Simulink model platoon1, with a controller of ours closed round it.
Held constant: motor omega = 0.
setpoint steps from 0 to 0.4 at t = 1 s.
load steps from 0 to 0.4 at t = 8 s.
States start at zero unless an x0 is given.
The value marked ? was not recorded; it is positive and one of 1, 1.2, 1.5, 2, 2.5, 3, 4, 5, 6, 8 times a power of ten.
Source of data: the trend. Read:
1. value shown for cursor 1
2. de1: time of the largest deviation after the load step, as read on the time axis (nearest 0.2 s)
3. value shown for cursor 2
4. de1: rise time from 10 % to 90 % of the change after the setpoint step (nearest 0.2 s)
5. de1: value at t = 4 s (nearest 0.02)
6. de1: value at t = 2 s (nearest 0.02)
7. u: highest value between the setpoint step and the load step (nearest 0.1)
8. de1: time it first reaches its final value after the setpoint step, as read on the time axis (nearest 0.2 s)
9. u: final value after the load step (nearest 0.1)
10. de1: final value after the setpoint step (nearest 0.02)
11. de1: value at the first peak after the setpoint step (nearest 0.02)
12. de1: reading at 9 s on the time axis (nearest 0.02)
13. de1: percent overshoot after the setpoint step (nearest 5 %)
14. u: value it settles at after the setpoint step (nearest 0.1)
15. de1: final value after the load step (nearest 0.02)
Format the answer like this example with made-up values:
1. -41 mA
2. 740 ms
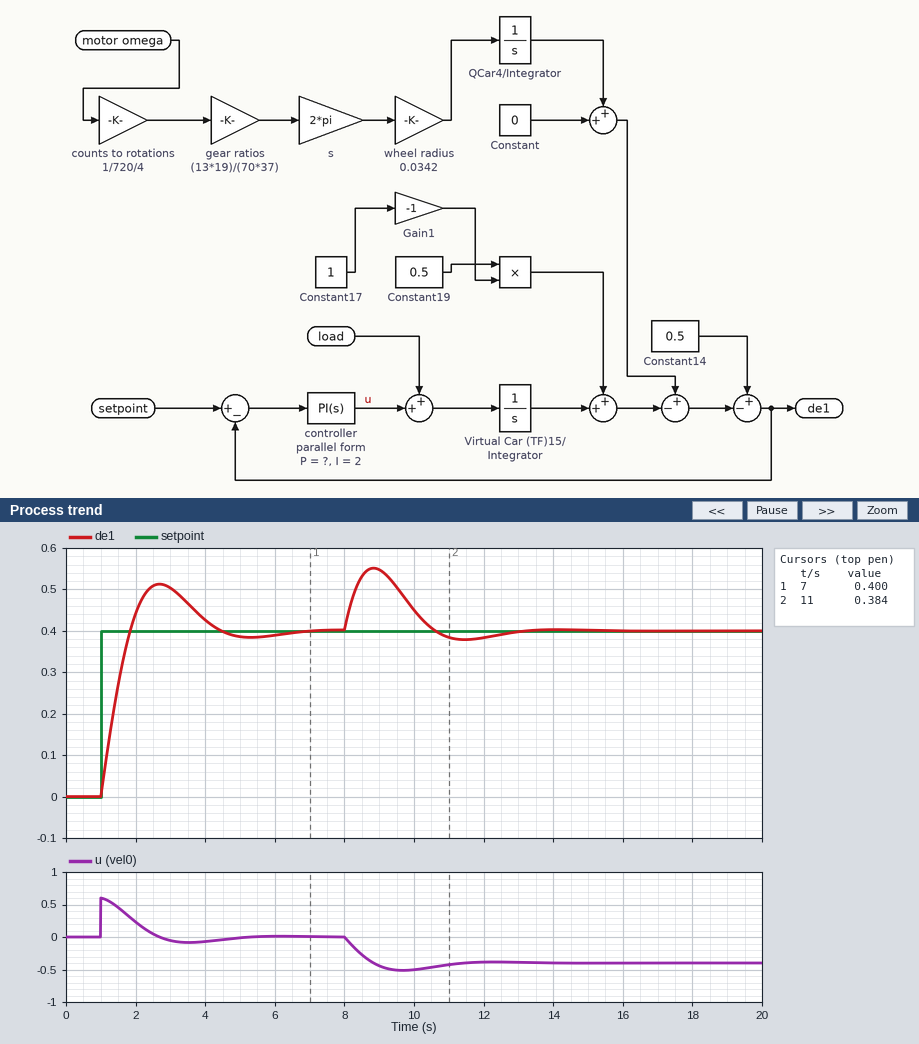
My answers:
1. 0.400
2. 8.8 s
3. 0.384
4. 0.6 s
5. 0.42
6. 0.44
7. 0.6
8. 1.8 s
9. -0.4
10. 0.40
11. 0.52
12. 0.54
13. 30 %
14. 0.0
15. 0.40
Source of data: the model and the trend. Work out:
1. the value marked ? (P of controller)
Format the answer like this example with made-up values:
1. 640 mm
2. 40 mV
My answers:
1. 1.5
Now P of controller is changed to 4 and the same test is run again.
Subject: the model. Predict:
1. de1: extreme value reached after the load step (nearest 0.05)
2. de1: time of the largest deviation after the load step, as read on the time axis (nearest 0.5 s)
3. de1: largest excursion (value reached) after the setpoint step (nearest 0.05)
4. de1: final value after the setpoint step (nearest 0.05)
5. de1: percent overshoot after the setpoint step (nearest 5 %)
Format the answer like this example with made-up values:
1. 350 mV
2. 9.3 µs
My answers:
1. 0.50
2. 8.5 s
3. 0.45
4. 0.40
5. 10 %
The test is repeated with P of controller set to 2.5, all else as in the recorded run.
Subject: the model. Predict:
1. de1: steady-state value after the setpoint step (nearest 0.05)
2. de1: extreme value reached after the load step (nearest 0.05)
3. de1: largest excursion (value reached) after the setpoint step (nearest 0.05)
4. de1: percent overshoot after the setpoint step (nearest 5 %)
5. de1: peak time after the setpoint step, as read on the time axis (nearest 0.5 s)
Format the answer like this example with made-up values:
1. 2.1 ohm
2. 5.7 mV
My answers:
1. 0.40
2. 0.50
3. 0.45
4. 15 %
5. 2.5 s
